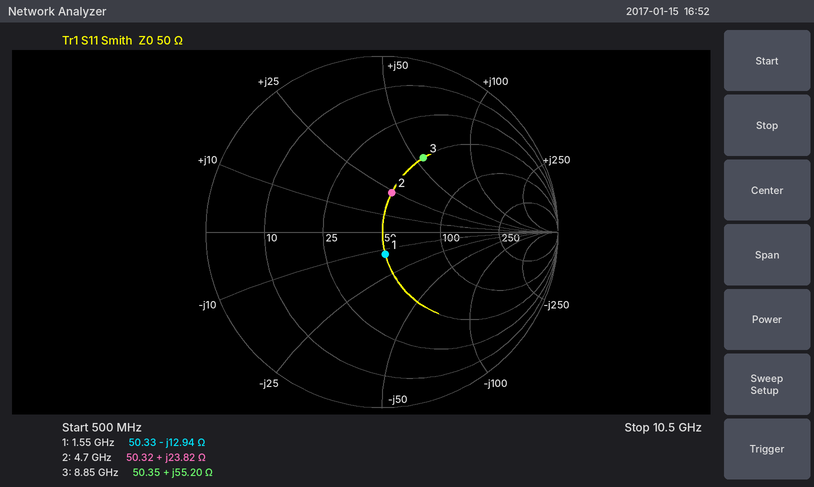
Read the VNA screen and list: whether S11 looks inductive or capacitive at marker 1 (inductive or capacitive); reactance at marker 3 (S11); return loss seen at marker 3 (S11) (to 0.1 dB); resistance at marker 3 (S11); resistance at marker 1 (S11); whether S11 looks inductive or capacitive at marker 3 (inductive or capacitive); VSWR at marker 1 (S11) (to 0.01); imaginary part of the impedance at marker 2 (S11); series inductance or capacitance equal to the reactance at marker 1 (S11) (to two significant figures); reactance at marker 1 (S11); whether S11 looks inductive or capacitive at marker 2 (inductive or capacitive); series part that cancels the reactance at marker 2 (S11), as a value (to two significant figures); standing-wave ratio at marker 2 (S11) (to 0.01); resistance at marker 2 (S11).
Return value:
capacitive
+55.20 Ω
6.3 dB
50.35 Ω
50.33 Ω
inductive
1.29
+23.82 Ω
7.9 pF
-12.94 Ω
inductive
1.4 pF
1.60
50.32 Ω
